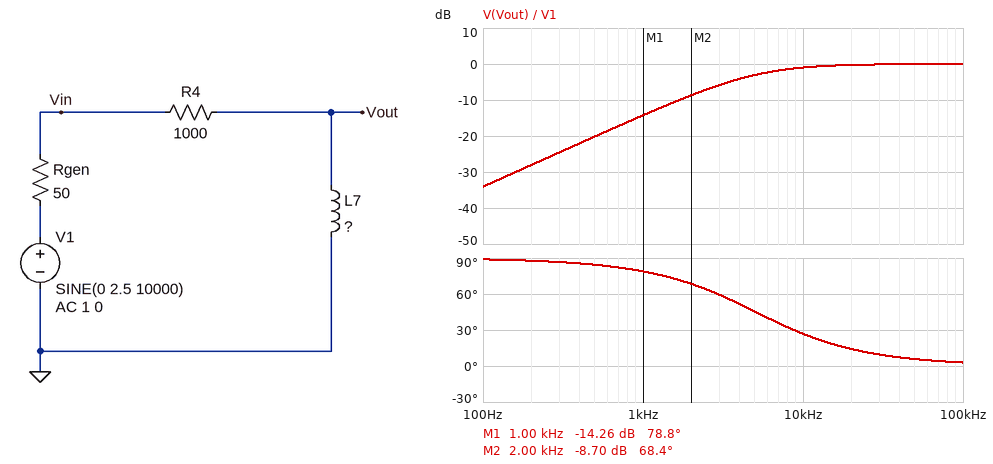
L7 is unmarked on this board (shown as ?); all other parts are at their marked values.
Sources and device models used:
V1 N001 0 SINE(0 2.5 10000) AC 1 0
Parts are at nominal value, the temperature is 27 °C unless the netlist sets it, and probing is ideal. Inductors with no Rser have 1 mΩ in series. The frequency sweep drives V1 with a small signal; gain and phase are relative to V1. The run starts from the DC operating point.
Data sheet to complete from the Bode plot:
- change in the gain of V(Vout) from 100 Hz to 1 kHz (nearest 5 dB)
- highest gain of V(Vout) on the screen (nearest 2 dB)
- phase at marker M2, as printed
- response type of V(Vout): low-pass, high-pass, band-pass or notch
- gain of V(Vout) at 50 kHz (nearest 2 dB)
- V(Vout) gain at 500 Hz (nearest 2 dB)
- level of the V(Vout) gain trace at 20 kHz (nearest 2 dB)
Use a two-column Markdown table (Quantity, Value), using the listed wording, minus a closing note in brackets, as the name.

| Quantity | Value |
|---|---|
| change in the gain of V(Vout) from 100 Hz to 1 kHz | 20 dB |
| highest gain of V(Vout) on the screen | 0 dB |
| phase at marker M2, as printed | 68.4 deg |
| response type of V(Vout): low-pass, high-pass, band-pass or notch | high-pass |
| gain of V(Vout) at 50 kHz | 0 dB |
| V(Vout) gain at 500 Hz | -20 dB |
| level of the V(Vout) gain trace at 20 kHz | 0 dB |
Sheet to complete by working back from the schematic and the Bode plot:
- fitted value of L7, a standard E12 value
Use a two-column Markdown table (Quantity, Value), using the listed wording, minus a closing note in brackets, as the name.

| Quantity | Value |
|---|---|
| fitted value of L7, a standard E12 value | 33 mH |
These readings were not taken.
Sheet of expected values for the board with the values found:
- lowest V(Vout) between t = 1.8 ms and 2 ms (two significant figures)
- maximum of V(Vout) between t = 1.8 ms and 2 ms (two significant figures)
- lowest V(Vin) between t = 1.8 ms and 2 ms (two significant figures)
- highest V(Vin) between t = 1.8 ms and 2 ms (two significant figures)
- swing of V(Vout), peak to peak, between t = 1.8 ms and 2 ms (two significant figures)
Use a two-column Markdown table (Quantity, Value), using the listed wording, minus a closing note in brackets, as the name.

| Quantity | Value |
|---|---|
| lowest V(Vout) between t = 1.8 ms and 2 ms | -2.2 V |
| maximum of V(Vout) between t = 1.8 ms and 2 ms | 2.2 V |
| lowest V(Vin) between t = 1.8 ms and 2 ms | -2.5 V |
| highest V(Vin) between t = 1.8 ms and 2 ms | 2.5 V |
| swing of V(Vout), peak to peak, between t = 1.8 ms and 2 ms | 4.5 V |
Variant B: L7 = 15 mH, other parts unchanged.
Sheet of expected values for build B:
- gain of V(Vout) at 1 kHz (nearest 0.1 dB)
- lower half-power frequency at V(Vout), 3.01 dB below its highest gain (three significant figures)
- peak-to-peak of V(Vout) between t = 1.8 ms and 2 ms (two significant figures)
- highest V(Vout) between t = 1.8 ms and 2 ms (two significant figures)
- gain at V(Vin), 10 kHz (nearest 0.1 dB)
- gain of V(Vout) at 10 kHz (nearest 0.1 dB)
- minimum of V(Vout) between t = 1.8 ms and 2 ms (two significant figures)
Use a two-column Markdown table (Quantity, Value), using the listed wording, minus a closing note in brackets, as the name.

| Quantity | Value |
|---|---|
| gain of V(Vout) at 1 kHz | -21.0 dB |
| lower half-power frequency at V(Vout), 3.01 dB below its highest gain | 11.1 kHz |
| peak-to-peak of V(Vout) between t = 1.8 ms and 2 ms | 3.3 V |
| highest V(Vout) between t = 1.8 ms and 2 ms | 1.7 V |
| gain at V(Vin), 10 kHz | -0.2 dB |
| gain of V(Vout) at 10 kHz | -3.5 dB |
| minimum of V(Vout) between t = 1.8 ms and 2 ms | -1.7 V |
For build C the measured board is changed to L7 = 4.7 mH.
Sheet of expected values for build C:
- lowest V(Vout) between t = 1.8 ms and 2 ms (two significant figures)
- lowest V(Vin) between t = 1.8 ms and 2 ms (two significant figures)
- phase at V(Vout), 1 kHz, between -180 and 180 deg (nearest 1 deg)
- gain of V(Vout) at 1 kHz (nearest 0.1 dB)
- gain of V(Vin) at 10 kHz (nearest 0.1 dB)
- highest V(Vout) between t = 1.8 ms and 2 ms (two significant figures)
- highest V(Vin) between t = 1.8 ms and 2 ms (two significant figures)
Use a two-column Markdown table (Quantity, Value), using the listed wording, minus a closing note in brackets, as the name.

| Quantity | Value |
|---|---|
| lowest V(Vout) between t = 1.8 ms and 2 ms | -680 mV |
| lowest V(Vin) between t = 1.8 ms and 2 ms | -2.4 V |
| phase at V(Vout), 1 kHz, between -180 and 180 deg | 88 deg |
| gain of V(Vout) at 1 kHz | -31.0 dB |
| gain of V(Vin) at 10 kHz | -0.4 dB |
| highest V(Vout) between t = 1.8 ms and 2 ms | 680 mV |
| highest V(Vin) between t = 1.8 ms and 2 ms | 2.4 V |
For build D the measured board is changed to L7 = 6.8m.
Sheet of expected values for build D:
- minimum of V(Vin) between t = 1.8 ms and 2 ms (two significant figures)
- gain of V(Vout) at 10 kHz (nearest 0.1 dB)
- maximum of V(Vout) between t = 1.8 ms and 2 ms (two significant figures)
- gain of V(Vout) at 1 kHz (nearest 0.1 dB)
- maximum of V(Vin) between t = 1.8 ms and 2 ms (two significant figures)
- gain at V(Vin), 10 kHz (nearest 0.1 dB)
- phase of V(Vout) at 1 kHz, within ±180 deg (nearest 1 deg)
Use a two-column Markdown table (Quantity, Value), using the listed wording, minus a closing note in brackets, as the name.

| Quantity | Value |
|---|---|
| minimum of V(Vin) between t = 1.8 ms and 2 ms | -2.4 V |
| gain of V(Vout) at 10 kHz | -8.5 dB |
| maximum of V(Vout) between t = 1.8 ms and 2 ms | 940 mV |
| gain of V(Vout) at 1 kHz | -27.8 dB |
| maximum of V(Vin) between t = 1.8 ms and 2 ms | 2.4 V |
| gain at V(Vin), 10 kHz | -0.4 dB |
| phase of V(Vout) at 1 kHz, within ±180 deg | 88 deg |
